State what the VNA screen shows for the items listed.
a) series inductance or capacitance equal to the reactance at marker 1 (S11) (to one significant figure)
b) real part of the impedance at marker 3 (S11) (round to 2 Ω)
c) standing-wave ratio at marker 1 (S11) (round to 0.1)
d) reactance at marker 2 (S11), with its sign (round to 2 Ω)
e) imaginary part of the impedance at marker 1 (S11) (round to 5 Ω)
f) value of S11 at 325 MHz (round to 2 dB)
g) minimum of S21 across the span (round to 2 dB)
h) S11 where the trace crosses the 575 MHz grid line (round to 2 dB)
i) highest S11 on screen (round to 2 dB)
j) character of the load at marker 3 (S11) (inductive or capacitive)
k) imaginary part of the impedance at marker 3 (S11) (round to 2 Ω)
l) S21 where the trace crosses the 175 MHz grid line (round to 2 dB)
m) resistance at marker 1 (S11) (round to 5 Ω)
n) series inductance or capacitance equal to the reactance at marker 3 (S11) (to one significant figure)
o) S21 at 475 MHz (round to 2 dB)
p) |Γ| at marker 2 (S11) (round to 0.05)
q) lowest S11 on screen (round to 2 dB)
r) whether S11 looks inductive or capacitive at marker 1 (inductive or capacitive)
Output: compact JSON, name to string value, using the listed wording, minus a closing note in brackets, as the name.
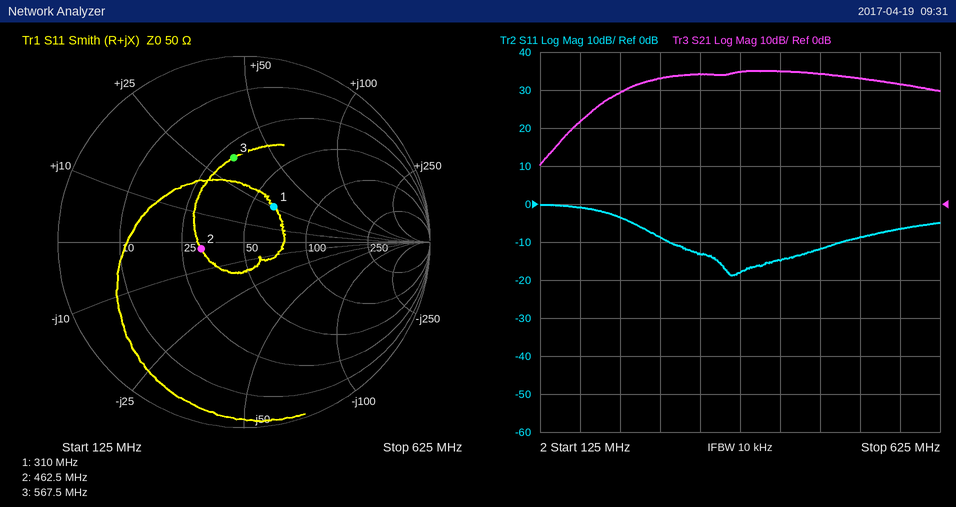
{"series inductance or capacitance equal to the reactance at marker 1 (S11)": "10 nH", "real part of the impedance at marker 3 (S11)": "30 Ω", "standing-wave ratio at marker 1 (S11)": "1.7", "reactance at marker 2 (S11), with its sign": "-2 Ω", "imaginary part of the impedance at marker 1 (S11)": "+25 Ω", "value of S11 at 325 MHz": "-14 dB", "minimum of S21 across the span": "10 dB", "S11 where the trace crosses the 575 MHz grid line": "-6 dB", "highest S11 on screen": "0 dB", "character of the load at marker 3 (S11)": "inductive", "imaginary part of the impedance at marker 3 (S11)": "+34 Ω", "S21 where the trace crosses the 175 MHz grid line": "22 dB", "resistance at marker 1 (S11)": "65 Ω", "series inductance or capacitance equal to the reactance at marker 3 (S11)": "10 nH", "S21 at 475 MHz": "34 dB", "|Γ| at marker 2 (S11)": "0.25", "lowest S11 on screen": "-18 dB", "whether S11 looks inductive or capacitive at marker 1": "inductive"}
